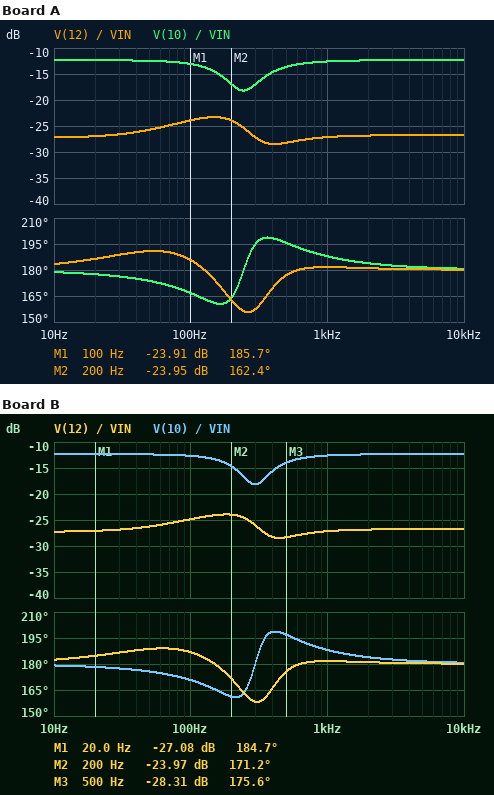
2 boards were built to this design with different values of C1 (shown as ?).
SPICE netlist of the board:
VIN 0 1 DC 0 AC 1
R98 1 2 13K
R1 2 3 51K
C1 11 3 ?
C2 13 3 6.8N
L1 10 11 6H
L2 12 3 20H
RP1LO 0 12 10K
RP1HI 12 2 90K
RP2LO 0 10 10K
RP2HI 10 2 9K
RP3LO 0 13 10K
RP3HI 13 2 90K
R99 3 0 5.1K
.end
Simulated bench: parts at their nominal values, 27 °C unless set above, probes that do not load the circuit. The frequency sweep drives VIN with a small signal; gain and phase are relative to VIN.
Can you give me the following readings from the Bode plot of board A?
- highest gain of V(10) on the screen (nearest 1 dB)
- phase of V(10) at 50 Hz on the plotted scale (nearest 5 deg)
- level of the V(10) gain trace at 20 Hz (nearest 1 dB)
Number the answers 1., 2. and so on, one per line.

1. -12 dB
2. 175 deg
3. -12 dB
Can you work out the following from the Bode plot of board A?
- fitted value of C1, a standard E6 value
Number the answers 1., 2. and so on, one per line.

1. 68 nF
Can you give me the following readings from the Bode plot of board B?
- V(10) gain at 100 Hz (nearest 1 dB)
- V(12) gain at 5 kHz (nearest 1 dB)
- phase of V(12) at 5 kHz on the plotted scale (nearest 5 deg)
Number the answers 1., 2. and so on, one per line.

1. -13 dB
2. -27 dB
3. 180 deg
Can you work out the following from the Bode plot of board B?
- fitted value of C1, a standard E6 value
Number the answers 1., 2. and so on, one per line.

1. 47 nF
